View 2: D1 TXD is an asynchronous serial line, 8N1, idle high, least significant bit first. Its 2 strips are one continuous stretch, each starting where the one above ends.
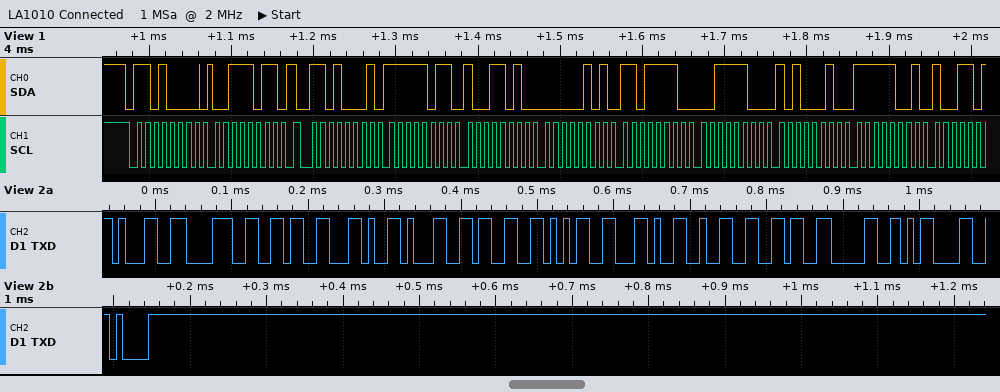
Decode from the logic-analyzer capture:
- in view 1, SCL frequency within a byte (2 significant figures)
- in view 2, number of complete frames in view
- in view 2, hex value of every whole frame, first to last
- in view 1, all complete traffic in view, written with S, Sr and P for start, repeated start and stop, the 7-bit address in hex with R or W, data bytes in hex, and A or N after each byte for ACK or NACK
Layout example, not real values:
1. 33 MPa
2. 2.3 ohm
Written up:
1. 100 kHz
2. 13
3. 31 38 36 2C 31 33 35 2C 32 36 30 0D 0A
4. S 68W A 3B A Sr 68R A FB A 9A A 05 A DE A 3C A A2 A F9 A
